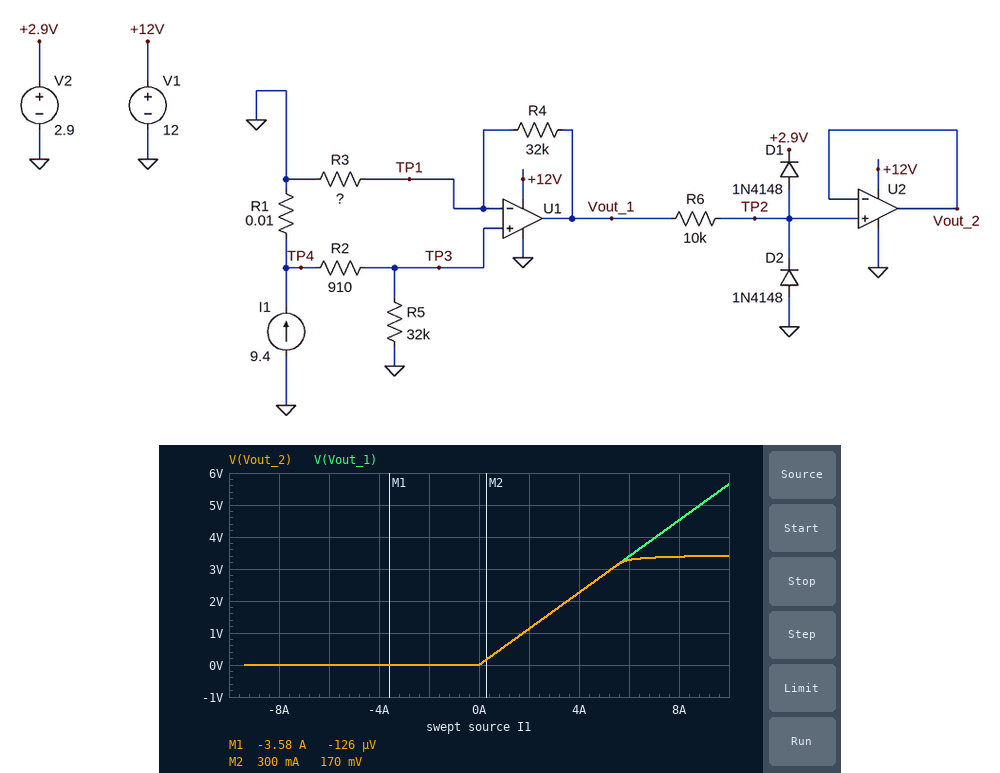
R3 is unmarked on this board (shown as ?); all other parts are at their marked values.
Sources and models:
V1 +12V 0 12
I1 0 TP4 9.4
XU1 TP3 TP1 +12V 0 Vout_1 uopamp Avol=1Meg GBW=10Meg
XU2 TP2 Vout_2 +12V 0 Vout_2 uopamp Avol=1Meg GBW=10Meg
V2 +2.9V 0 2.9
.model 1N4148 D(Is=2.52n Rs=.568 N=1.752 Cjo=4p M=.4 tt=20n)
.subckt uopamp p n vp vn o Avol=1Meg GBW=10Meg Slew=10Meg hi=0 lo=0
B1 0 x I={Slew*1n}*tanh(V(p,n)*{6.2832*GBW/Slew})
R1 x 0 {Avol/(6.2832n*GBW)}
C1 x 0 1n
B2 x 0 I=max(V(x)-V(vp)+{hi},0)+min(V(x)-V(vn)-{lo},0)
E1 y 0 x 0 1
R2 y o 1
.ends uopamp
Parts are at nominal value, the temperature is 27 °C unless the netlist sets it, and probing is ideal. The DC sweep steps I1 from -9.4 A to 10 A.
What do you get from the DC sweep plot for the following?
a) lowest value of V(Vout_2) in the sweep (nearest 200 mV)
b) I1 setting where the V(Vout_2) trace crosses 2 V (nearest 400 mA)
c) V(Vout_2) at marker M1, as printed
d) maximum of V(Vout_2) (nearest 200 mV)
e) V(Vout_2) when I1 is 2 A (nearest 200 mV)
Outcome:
0 V
3.6 A
-126 µV
3.4 V
1.2 V
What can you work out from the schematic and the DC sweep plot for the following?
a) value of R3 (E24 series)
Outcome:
560 Ω
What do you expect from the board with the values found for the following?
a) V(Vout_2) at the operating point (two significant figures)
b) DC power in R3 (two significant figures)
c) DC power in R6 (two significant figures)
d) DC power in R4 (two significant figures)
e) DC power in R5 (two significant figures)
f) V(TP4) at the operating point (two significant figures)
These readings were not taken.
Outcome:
3.4 V
15 µW
360 µW
850 µW
260 nW
94 mV
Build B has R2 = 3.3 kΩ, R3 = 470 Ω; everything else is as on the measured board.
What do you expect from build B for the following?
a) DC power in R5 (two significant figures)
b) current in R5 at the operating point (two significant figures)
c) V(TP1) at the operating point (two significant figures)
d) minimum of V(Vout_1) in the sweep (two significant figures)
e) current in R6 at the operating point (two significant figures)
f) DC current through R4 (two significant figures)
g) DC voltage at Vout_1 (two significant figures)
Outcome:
230 nW
2.7 µA
85 mV
-4.9 mV
250 µA
180 µA
5.9 V
